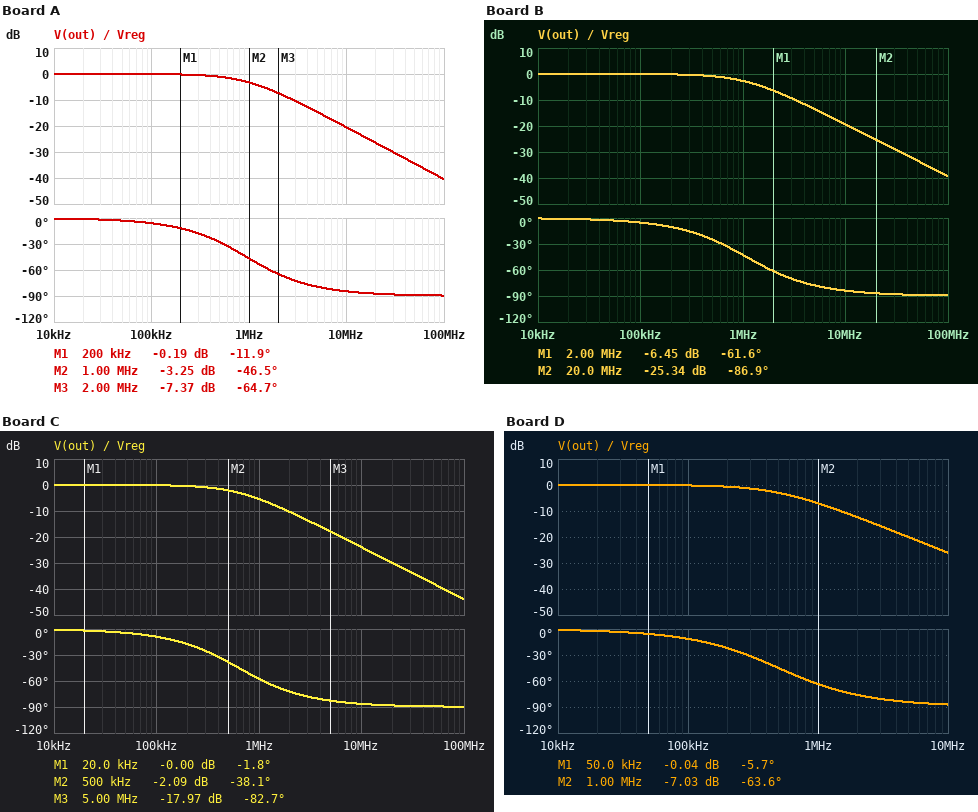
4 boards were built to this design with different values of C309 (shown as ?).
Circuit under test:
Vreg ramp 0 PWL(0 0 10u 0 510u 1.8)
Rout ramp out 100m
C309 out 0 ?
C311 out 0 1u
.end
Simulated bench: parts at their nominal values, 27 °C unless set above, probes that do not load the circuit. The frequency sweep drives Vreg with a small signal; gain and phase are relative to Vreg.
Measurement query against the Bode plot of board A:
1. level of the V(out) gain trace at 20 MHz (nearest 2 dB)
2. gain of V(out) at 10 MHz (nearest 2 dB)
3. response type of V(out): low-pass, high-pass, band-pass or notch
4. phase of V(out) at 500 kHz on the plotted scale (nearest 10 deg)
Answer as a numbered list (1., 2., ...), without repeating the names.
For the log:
1. -26 dB
2. -20 dB
3. low-pass
4. -30 deg
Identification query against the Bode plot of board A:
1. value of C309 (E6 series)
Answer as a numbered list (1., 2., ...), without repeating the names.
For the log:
1. 680 nF
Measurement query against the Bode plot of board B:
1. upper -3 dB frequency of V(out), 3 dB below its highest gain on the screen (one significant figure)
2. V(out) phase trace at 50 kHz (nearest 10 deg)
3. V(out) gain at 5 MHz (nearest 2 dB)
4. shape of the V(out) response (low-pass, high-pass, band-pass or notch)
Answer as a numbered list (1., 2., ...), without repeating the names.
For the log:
1. 1 MHz
2. 0 deg
3. -14 dB
4. low-pass
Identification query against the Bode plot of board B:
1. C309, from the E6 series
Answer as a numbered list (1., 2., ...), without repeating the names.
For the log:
1. 470 nF
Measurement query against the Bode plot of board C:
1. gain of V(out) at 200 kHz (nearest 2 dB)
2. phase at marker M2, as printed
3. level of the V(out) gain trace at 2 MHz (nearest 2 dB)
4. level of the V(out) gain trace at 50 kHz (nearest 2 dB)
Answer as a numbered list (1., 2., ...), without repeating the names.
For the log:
1. 0 dB
2. -38.1 deg
3. -10 dB
4. 0 dB
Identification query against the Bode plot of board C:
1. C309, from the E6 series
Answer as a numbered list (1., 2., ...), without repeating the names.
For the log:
1. 1.5 µF
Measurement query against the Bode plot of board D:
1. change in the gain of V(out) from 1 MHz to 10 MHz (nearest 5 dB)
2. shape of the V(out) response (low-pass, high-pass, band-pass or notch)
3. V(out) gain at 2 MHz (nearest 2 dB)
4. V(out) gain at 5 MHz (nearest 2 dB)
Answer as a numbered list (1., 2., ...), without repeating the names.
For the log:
1. -20 dB
2. low-pass
3. -12 dB
4. -20 dB
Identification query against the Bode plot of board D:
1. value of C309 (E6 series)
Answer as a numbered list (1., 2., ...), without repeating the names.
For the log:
1. 2.2 µF
